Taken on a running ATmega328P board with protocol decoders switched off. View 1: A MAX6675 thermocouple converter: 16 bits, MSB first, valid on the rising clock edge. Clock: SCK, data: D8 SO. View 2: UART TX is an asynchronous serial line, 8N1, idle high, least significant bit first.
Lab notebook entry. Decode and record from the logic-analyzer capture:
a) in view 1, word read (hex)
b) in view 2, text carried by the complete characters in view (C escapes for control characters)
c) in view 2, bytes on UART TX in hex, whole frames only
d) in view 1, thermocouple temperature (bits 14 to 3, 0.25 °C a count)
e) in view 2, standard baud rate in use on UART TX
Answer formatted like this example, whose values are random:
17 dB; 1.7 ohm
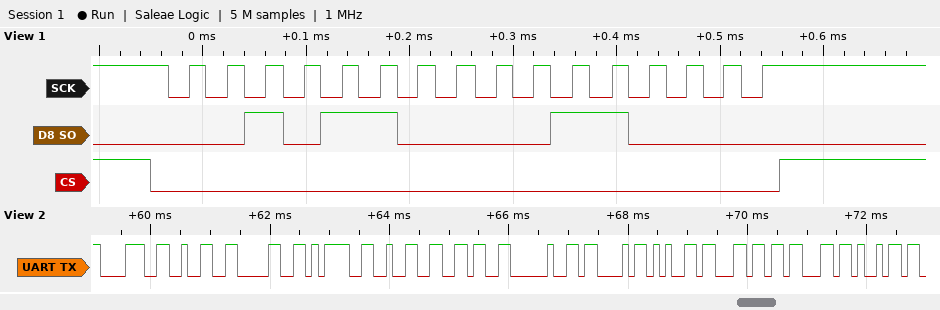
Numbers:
0x2C30; "820=26 Celci"; 0x38 0x32 0x30 0x3D 0x32 0x36 0x20 0x43 0x65 0x6C 0x63 0x69; 353.50 °C; 9600 baud
